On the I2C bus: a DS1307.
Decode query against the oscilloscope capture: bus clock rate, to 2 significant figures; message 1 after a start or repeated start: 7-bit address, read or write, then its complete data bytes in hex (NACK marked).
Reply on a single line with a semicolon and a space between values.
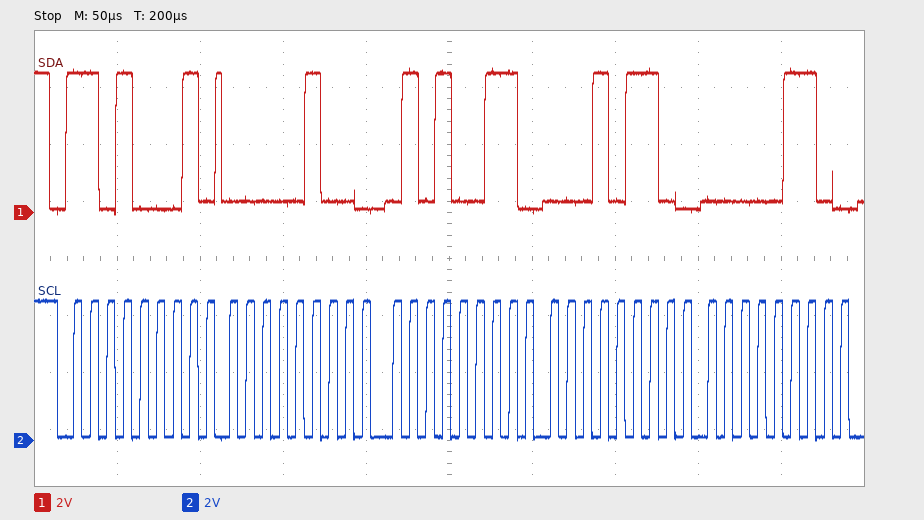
100 kHz; 0x68 read: 04 53 16 06
